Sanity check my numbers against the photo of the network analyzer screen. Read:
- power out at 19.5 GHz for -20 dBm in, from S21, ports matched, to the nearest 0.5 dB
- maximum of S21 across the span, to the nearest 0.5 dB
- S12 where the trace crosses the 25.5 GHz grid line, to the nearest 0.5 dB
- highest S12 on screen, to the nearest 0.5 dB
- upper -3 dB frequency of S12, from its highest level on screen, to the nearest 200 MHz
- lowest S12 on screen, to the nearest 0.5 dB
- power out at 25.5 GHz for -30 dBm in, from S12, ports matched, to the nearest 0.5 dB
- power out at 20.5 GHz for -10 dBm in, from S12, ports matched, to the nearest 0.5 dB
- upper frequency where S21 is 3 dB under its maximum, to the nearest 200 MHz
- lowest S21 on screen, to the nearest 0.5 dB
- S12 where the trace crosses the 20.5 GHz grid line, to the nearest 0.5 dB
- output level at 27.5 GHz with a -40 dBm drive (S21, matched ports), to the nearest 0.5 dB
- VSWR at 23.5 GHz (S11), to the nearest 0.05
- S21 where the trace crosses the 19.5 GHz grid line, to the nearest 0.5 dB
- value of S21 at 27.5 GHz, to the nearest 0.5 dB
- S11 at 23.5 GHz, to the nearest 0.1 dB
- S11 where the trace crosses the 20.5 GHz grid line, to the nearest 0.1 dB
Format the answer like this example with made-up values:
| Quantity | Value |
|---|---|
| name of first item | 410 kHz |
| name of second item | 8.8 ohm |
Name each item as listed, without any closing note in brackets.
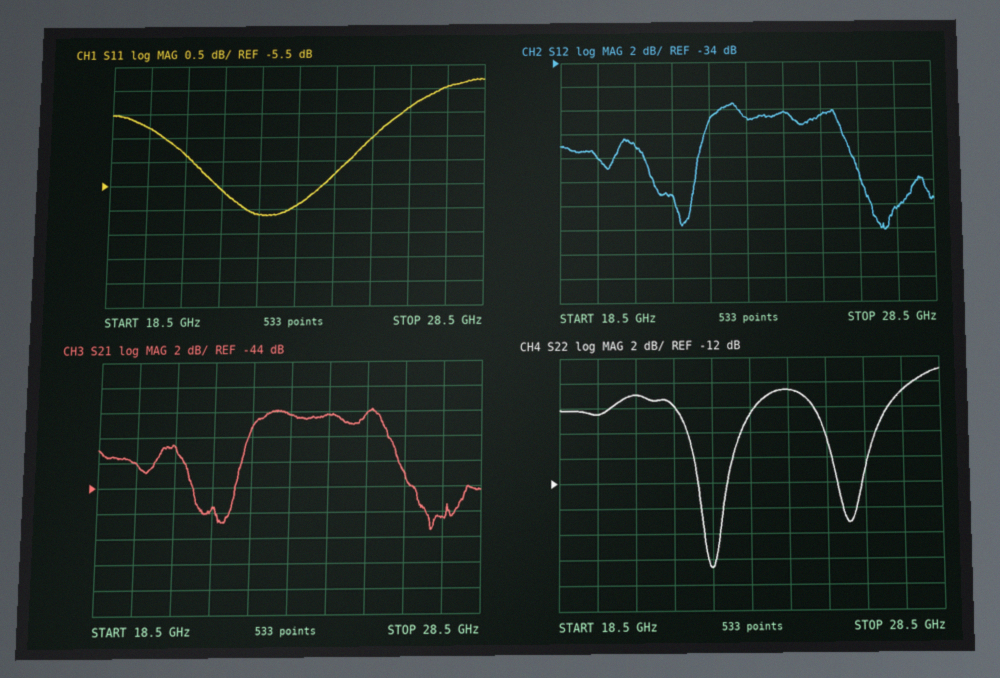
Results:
| Quantity | Value |
|---|---|
| power out at 19.5 GHz for -20 dBm in, from S21, ports matched, to the nearest 0.5 dB | -62.0 dBm |
| maximum of S21 across the span, to the nearest 0.5 dB | -38.0 dB |
| S12 where the trace crosses the 25.5 GHz grid line, to the nearest 0.5 dB | -38.5 dB |
| highest S12 on screen, to the nearest 0.5 dB | -37.5 dB |
| upper -3 dB frequency of S12, from its highest level on screen, to the nearest 200 MHz | 26.2 GHz |
| lowest S12 on screen, to the nearest 0.5 dB | -48.0 dB |
| power out at 25.5 GHz for -30 dBm in, from S12, ports matched, to the nearest 0.5 dB | -68.5 dBm |
| power out at 20.5 GHz for -10 dBm in, from S12, ports matched, to the nearest 0.5 dB | -51.0 dBm |
| upper frequency where S21 is 3 dB under its maximum, to the nearest 200 MHz | 26.2 GHz |
| lowest S21 on screen, to the nearest 0.5 dB | -47.5 dB |
| S12 where the trace crosses the 20.5 GHz grid line, to the nearest 0.5 dB | -41.0 dB |
| output level at 27.5 GHz with a -40 dBm drive (S21, matched ports), to the nearest 0.5 dB | -86.5 dBm |
| VSWR at 23.5 GHz (S11), to the nearest 0.05 | 3.05 |
| S21 where the trace crosses the 19.5 GHz grid line, to the nearest 0.5 dB | -42.0 dB |
| value of S21 at 27.5 GHz, to the nearest 0.5 dB | -46.5 dB |
| S11 at 23.5 GHz, to the nearest 0.1 dB | -5.9 dB |
| S11 where the trace crosses the 20.5 GHz grid line, to the nearest 0.1 dB | -4.9 dB |
